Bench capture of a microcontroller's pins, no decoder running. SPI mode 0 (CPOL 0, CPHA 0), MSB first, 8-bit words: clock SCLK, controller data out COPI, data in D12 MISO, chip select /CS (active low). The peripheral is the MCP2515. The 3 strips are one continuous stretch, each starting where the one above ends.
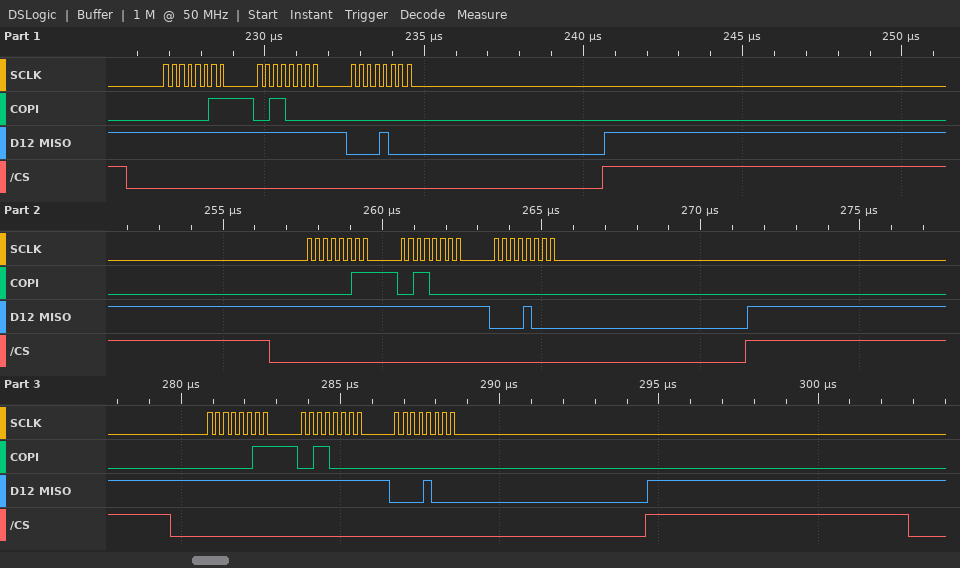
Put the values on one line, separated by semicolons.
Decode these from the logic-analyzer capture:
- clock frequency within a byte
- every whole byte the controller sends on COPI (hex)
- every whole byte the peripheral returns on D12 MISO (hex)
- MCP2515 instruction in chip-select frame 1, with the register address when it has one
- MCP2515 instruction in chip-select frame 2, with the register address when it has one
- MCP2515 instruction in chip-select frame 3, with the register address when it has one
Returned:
4 MHz; 03 30 00 03 30 00 03 30 00; FF FF 08 FF FF 08 FF FF 08; READ 0x30; READ 0x30; READ 0x30
